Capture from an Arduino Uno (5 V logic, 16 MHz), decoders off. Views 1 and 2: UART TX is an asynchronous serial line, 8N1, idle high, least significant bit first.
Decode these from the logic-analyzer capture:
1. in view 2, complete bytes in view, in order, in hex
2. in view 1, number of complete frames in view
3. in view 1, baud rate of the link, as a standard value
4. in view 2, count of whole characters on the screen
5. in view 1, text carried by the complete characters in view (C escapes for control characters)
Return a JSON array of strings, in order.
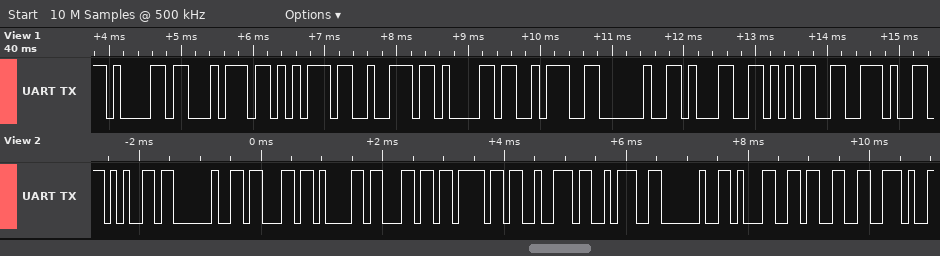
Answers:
["0x65 0x20 0x63 0x61 0x6C 0x6F 0x72 0x3A 0x20 0x31 0x33 0x2E", "10", "9600 baud", "12", "\"atura: 15.\""]
